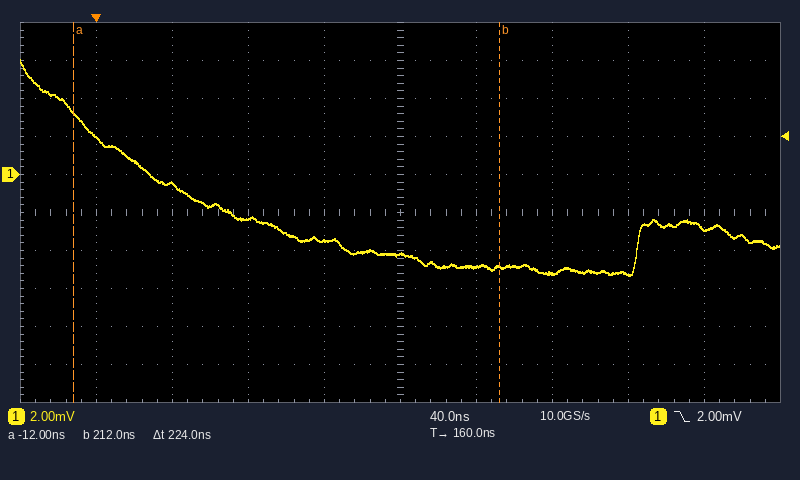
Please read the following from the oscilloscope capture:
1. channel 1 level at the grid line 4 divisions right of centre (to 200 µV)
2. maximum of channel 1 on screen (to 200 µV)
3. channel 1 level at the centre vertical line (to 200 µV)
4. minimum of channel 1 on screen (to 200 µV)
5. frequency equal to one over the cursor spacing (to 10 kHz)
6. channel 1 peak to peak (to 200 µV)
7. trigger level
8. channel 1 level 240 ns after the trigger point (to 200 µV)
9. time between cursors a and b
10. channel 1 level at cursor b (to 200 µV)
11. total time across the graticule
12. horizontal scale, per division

-2.8 mV
6.0 mV
-4.2 mV
-5.4 mV
4.46 MHz
11.4 mV
2.00 mV
-5.2 mV
224 ns
-4.8 mV
400 ns
40 ns
